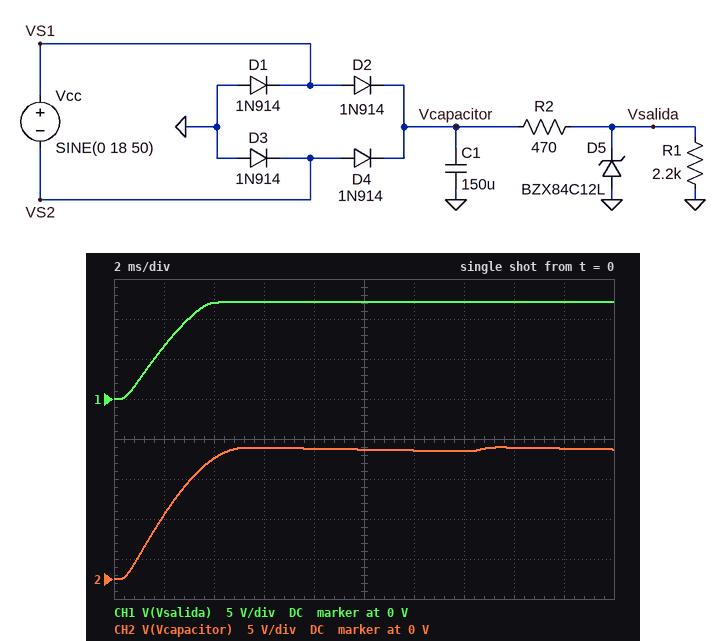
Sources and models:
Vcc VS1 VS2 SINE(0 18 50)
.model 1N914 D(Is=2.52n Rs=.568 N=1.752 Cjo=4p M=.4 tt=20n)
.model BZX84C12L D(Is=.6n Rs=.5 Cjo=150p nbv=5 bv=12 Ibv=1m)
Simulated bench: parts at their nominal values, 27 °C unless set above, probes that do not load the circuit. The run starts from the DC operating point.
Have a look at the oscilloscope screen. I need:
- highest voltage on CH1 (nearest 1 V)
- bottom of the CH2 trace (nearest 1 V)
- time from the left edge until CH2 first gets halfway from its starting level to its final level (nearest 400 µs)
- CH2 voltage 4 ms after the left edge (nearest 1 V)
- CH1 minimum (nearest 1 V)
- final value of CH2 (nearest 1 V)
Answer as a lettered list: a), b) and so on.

a) 12 V
b) 0 V
c) 2.0 ms
d) 15 V
e) 0 V
f) 16 V
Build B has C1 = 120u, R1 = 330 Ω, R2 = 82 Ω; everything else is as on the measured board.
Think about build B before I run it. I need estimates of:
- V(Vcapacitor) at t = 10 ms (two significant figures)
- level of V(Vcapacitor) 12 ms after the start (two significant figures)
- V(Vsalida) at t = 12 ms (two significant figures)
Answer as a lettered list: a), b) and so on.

a) 15 V
b) 14 V
c) 11 V
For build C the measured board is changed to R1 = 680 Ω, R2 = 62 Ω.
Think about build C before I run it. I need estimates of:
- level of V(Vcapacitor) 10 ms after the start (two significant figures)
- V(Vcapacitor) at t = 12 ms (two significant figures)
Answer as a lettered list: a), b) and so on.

a) 15 V
b) 14 V
